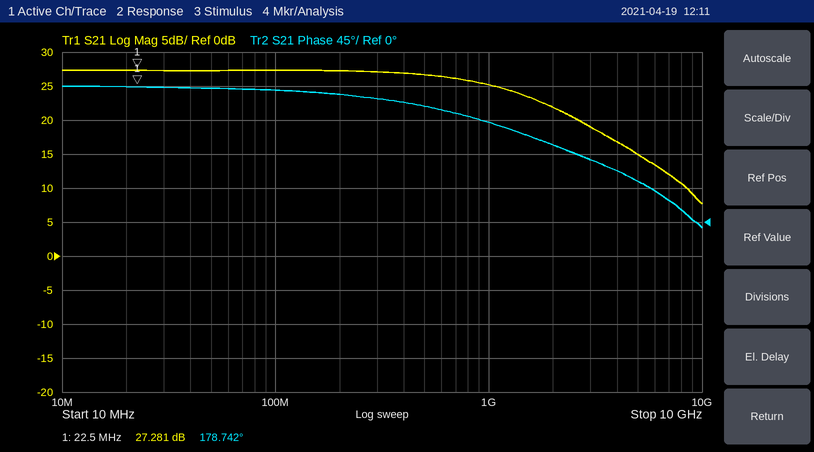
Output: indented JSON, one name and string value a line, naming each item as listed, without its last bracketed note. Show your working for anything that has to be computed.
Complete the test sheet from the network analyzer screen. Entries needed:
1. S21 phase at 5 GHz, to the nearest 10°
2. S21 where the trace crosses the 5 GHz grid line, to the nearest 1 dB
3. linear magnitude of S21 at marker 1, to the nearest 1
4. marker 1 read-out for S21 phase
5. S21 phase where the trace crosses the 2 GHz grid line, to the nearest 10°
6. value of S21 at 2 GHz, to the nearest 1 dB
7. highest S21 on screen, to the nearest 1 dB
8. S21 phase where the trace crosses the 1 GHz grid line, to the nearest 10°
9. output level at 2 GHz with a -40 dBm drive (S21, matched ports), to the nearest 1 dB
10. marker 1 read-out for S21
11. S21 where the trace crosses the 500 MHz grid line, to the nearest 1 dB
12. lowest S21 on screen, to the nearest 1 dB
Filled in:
{
  "S21 phase at 5 GHz, to the nearest 10°": "50°",
  "S21 where the trace crosses the 5 GHz grid line, to the nearest 1 dB": "15 dB",
  "linear magnitude of S21 at marker 1, to the nearest 1": "10^(27.281/20) ≈ 23",
  "marker 1 read-out for S21 phase": "178.742°",
  "S21 phase where the trace crosses the 2 GHz grid line, to the nearest 10°": "100°",
  "value of S21 at 2 GHz, to the nearest 1 dB": "22 dB",
  "highest S21 on screen, to the nearest 1 dB": "27 dB",
  "S21 phase where the trace crosses the 1 GHz grid line, to the nearest 10°": "130°",
  "output level at 2 GHz with a -40 dBm drive (S21, matched ports), to the nearest 1 dB": "-40 dBm + (22 dB) = -18 dBm",
  "marker 1 read-out for S21": "27.281 dB",
  "S21 where the trace crosses the 500 MHz grid line, to the nearest 1 dB": "27 dB",
  "lowest S21 on screen, to the nearest 1 dB": "8 dB"
}
